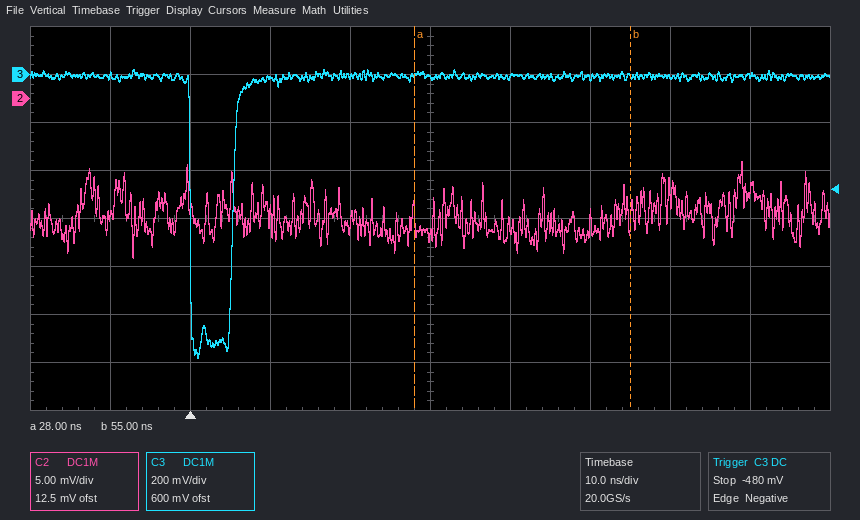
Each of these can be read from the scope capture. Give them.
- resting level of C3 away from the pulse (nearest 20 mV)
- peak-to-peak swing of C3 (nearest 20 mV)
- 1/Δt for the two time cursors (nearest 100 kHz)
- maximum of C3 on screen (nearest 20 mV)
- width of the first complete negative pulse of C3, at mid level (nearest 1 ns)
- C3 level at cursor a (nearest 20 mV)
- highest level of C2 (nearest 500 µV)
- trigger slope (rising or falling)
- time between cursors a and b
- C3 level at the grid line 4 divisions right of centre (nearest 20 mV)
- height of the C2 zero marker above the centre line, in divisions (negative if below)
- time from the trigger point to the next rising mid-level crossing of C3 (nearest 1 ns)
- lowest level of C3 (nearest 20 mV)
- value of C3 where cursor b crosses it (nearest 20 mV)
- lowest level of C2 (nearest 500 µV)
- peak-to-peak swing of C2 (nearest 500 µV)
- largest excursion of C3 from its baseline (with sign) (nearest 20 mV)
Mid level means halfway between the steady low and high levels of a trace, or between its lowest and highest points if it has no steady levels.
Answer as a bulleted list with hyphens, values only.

- 0 mV
- 1.20 V
- 37.0 MHz
- 20 mV
- 5 ns
- 0 mV
- -6.5 mV
- falling
- 27 ns
- 0 mV
- +2.5 div
- 5 ns
- -1.18 V
- 0 mV
- -16.5 mV
- 10.0 mV
- -1.18 V
